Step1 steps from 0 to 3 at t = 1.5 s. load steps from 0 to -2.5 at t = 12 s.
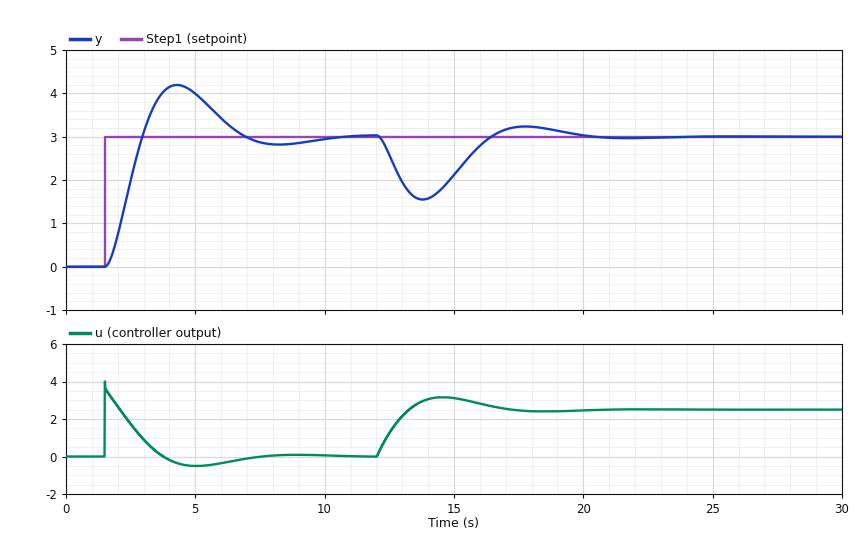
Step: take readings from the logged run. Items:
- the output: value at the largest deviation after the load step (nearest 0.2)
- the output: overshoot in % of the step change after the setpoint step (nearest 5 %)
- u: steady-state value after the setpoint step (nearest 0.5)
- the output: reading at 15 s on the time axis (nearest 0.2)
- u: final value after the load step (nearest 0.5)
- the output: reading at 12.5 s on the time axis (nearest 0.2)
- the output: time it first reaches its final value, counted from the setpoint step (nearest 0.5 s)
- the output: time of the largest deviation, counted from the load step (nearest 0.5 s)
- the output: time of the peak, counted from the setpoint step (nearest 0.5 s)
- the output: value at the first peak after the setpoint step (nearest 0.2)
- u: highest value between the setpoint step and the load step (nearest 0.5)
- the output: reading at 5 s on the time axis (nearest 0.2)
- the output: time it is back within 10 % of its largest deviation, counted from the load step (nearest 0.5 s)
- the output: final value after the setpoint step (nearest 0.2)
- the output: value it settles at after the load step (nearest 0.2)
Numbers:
1.6
40 %
0.0
2.2
2.5
2.6
1.5 s
2.0 s
3.0 s
4.2
4.0
4.0
7.0 s
3.0
3.0
